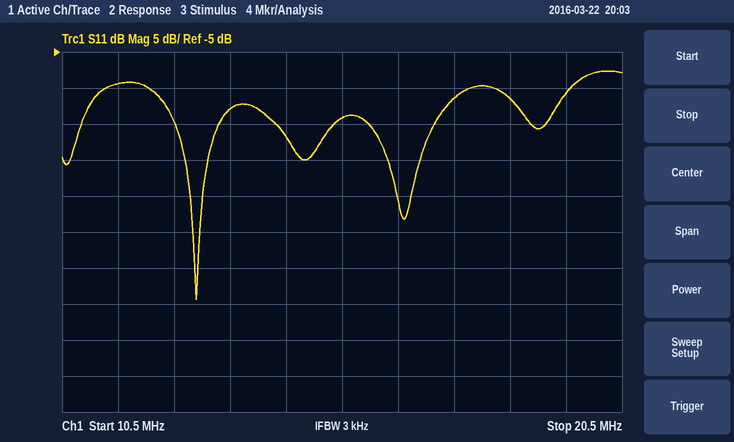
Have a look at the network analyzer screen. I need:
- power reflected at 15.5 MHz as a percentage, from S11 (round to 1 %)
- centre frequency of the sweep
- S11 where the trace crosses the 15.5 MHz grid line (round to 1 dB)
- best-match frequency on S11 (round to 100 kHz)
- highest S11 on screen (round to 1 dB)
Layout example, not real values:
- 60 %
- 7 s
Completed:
- 4 %
- 15.5 MHz
- -14 dB
- 12.9 MHz
- -8 dB
